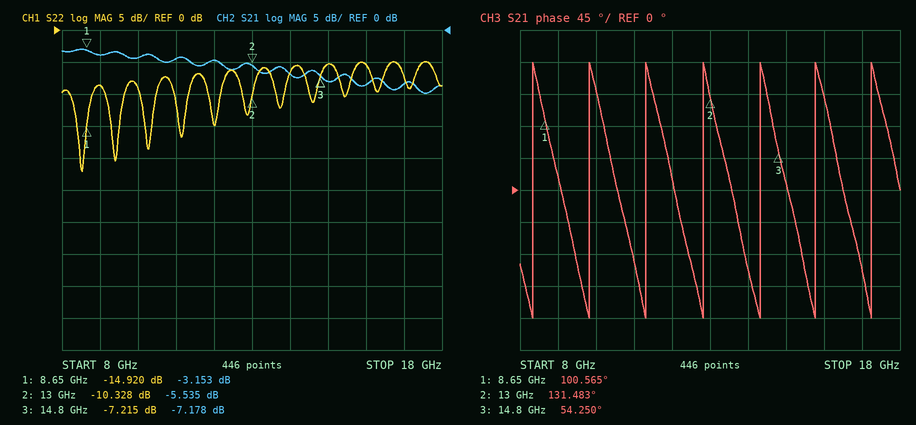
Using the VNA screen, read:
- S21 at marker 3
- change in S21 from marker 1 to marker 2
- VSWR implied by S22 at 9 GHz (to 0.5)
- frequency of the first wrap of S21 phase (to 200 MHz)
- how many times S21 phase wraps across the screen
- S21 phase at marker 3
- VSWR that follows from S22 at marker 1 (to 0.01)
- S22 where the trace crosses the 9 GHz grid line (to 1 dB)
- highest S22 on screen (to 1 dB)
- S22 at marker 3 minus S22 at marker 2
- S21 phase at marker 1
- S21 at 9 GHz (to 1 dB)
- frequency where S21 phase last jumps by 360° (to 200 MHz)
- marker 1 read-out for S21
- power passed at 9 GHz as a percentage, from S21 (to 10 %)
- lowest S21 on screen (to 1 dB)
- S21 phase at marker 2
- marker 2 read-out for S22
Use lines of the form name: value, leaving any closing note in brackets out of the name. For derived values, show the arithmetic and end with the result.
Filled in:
S21 at marker 3: -7.178 dB
change in S21 from marker 1 to marker 2: -5.535 − (-3.153) = -2.382 dB
VSWR implied by S22 at 9 GHz: |Γ| = 10^(-9/20) = 0.3548; VSWR = (1 + 0.3548)/(1 − 0.3548) ≈ 2.10, so 2.0 to the nearest 0.5
frequency of the first wrap of S21 phase: 8.4 GHz
how many times S21 phase wraps across the screen: 7
S21 phase at marker 3: 54.250°
VSWR that follows from S22 at marker 1: (1 + 0.1795)/(1 − 0.1795) ≈ 1.44
S22 where the trace crosses the 9 GHz grid line: -9 dB
highest S22 on screen: -5 dB
S22 at marker 3 minus S22 at marker 2: -7.215 − (-10.328) = 3.113 dB
S21 phase at marker 1: 100.565°
S21 at 9 GHz: -4 dB
frequency where S21 phase last jumps by 360°: 17.2 GHz
marker 1 read-out for S21: -3.153 dB
power passed at 9 GHz as a percentage, from S21: 10^(-4/10) ≈ 40 %
lowest S21 on screen: -10 dB
S21 phase at marker 2: 131.483°
marker 2 read-out for S22: -10.328 dB
